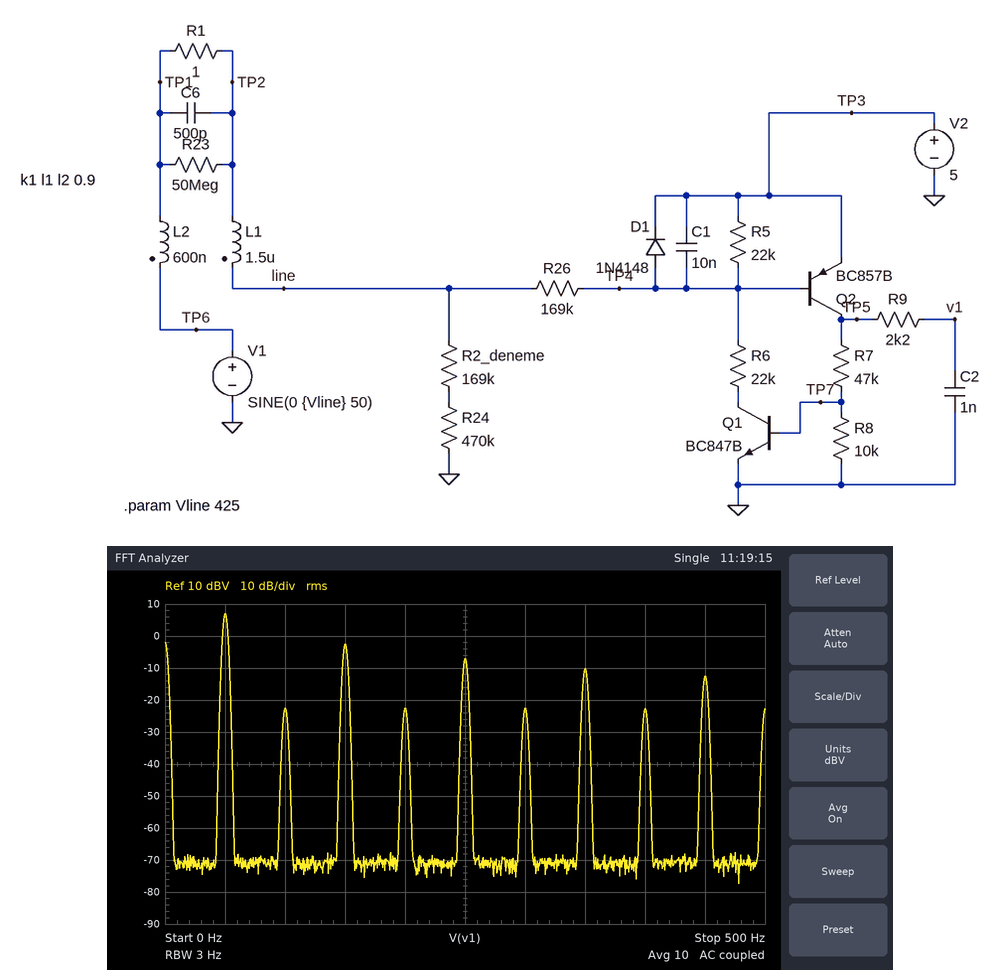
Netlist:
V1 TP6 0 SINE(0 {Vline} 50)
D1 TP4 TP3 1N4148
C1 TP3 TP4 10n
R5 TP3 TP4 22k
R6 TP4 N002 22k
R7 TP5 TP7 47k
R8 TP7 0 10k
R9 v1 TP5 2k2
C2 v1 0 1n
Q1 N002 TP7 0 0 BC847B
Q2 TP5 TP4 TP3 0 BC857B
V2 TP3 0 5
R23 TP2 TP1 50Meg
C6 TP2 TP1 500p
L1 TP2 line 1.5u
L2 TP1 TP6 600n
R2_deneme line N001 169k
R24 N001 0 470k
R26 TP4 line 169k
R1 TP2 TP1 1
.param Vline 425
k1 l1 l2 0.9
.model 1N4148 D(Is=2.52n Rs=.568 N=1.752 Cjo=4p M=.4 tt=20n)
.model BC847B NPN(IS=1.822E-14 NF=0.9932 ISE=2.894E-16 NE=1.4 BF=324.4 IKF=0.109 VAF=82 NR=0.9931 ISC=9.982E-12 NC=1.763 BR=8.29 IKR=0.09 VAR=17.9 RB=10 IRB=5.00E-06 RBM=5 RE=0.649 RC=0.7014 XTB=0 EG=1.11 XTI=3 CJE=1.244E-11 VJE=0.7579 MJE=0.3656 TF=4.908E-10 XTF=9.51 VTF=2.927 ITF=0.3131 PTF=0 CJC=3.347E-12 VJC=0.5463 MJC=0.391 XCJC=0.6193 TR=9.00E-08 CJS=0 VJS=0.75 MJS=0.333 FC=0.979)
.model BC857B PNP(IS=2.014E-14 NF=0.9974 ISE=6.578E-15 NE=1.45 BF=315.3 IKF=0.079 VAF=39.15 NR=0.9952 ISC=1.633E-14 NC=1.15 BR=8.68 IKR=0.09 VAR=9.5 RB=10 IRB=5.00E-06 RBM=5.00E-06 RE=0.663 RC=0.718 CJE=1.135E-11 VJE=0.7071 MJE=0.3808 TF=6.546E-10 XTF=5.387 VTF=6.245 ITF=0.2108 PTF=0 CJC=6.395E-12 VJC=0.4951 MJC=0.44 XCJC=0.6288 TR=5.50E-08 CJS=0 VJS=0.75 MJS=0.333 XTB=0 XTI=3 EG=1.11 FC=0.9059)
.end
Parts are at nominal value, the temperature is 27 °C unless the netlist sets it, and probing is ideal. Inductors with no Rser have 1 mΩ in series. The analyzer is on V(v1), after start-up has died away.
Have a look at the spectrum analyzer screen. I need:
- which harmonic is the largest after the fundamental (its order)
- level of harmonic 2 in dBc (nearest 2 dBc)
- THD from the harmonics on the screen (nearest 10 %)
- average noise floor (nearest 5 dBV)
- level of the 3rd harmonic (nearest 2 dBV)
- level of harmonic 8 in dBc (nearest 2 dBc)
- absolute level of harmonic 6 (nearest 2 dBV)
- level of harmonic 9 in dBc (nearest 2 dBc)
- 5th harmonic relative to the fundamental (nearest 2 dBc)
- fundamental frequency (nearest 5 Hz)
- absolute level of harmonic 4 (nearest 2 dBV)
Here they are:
3
-30 dBc
40 %
-70 dBV
-2 dBV
-30 dBc
-22 dBV
-20 dBc
-14 dBc
50 Hz
-22 dBV
